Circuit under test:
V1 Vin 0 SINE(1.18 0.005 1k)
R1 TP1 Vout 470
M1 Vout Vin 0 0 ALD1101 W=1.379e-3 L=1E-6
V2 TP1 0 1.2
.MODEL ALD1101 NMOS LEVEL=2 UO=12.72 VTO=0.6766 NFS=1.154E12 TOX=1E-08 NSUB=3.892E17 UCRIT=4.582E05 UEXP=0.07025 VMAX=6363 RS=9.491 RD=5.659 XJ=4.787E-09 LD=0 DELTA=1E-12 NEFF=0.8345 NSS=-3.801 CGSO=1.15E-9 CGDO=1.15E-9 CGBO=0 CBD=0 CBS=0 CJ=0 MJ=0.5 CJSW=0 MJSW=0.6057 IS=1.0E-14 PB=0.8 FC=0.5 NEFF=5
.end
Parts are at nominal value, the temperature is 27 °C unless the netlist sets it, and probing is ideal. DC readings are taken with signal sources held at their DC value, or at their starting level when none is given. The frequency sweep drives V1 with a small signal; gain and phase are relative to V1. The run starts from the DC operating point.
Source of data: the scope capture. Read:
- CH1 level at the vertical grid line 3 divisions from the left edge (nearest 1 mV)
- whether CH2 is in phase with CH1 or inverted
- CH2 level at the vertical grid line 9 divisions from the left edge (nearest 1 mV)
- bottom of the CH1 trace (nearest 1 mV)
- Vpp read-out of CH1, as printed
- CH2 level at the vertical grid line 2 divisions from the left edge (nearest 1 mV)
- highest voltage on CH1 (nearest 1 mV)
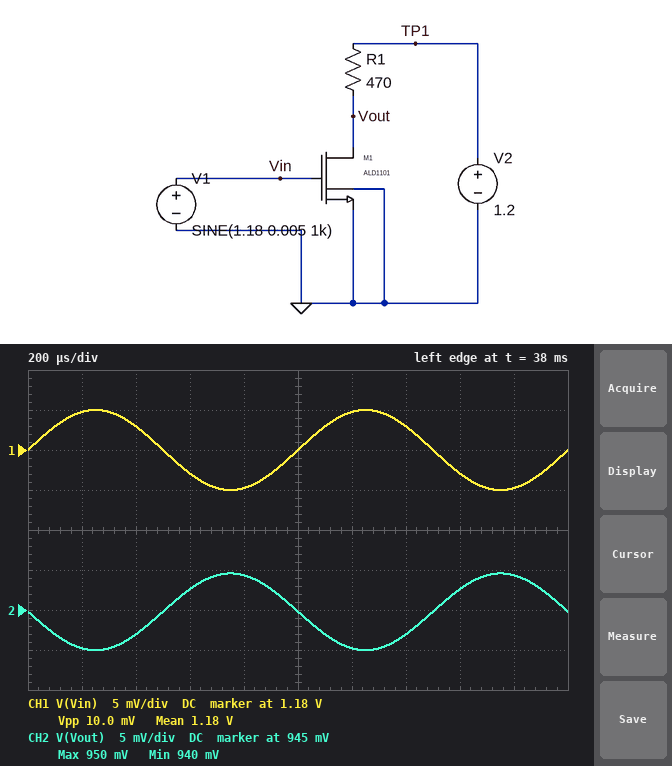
1.177 V
inverted
949 mV
1.175 V
10.0 mV
942 mV
1.185 V
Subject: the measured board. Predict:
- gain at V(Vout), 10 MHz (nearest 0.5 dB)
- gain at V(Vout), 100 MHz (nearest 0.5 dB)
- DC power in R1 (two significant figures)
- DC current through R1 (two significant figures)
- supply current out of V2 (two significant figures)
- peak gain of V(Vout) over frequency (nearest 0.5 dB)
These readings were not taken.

-0.5 dB
0 dB
140 µW
540 µA
540 µA
0.5 dB
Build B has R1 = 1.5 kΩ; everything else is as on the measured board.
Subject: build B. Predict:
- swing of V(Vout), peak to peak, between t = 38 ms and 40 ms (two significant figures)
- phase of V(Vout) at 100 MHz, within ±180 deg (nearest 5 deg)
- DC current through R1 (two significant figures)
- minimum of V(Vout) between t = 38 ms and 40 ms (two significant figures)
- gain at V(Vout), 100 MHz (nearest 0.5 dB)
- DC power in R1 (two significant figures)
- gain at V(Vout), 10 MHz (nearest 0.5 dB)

29 mV
95 deg
530 µA
390 mV
5.5 dB
430 µW
9.0 dB
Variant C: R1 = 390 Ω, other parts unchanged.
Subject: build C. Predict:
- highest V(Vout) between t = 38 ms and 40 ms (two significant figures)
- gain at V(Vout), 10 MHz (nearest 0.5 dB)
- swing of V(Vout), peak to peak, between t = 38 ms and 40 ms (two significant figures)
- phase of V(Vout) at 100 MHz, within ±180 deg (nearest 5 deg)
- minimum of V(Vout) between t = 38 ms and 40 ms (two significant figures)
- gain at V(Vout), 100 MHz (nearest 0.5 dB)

990 mV
-2.0 dB
8.0 mV
130 deg
980 mV
-1.5 dB
